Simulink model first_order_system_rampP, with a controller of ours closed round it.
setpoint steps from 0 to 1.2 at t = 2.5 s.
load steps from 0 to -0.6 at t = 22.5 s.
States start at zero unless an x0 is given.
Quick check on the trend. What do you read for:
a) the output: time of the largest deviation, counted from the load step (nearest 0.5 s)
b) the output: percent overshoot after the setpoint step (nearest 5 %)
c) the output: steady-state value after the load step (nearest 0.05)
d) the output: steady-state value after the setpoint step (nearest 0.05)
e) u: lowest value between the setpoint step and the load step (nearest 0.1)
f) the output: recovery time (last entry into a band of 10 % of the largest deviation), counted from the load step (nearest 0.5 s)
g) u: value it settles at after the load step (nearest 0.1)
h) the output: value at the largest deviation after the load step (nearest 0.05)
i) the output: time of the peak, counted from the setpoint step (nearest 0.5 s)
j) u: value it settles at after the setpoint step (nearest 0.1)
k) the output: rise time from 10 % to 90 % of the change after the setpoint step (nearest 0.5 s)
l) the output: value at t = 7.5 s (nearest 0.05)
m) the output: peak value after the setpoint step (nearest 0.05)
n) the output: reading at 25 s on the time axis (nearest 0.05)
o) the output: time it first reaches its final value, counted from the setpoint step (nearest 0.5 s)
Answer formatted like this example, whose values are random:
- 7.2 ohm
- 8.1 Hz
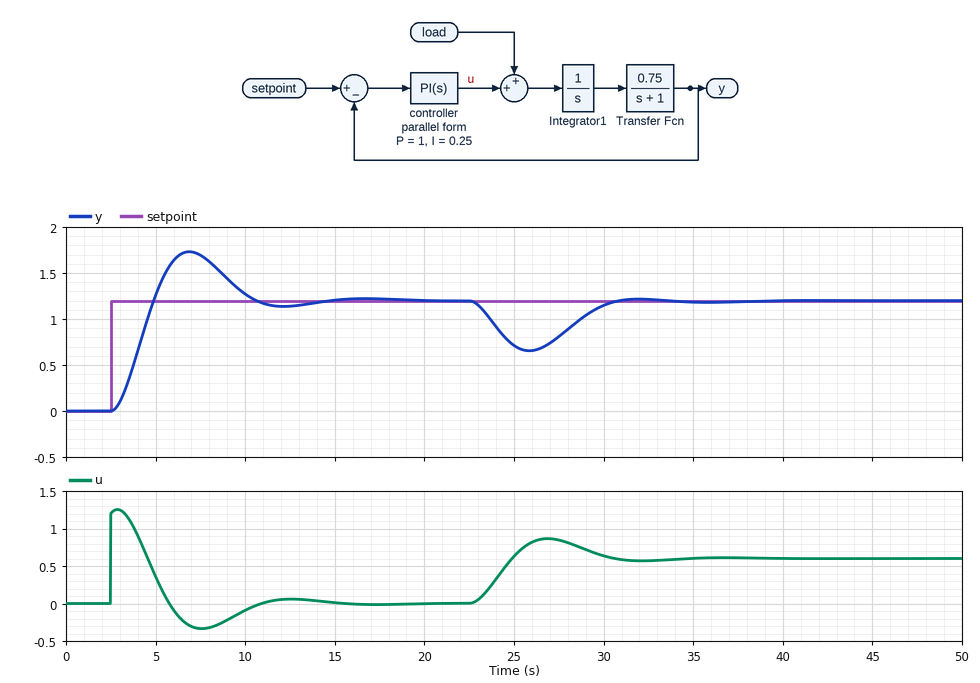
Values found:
- 3.5 s
- 45 %
- 1.20
- 1.20
- -0.3
- 7.5 s
- 0.6
- 0.65
- 4.5 s
- 0.0
- 1.5 s
- 1.70
- 1.75
- 0.70
- 2.5 s
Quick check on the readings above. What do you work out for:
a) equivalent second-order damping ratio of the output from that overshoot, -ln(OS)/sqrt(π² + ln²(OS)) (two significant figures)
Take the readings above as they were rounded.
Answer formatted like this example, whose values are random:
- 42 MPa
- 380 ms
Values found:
- 0.25
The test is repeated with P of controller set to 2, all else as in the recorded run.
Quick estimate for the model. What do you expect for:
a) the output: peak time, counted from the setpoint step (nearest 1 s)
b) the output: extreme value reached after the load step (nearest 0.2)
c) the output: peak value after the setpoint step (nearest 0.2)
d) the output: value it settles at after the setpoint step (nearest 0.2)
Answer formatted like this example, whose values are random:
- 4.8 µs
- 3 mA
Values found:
- 3 s
- 0.8
- 1.6
- 1.2
